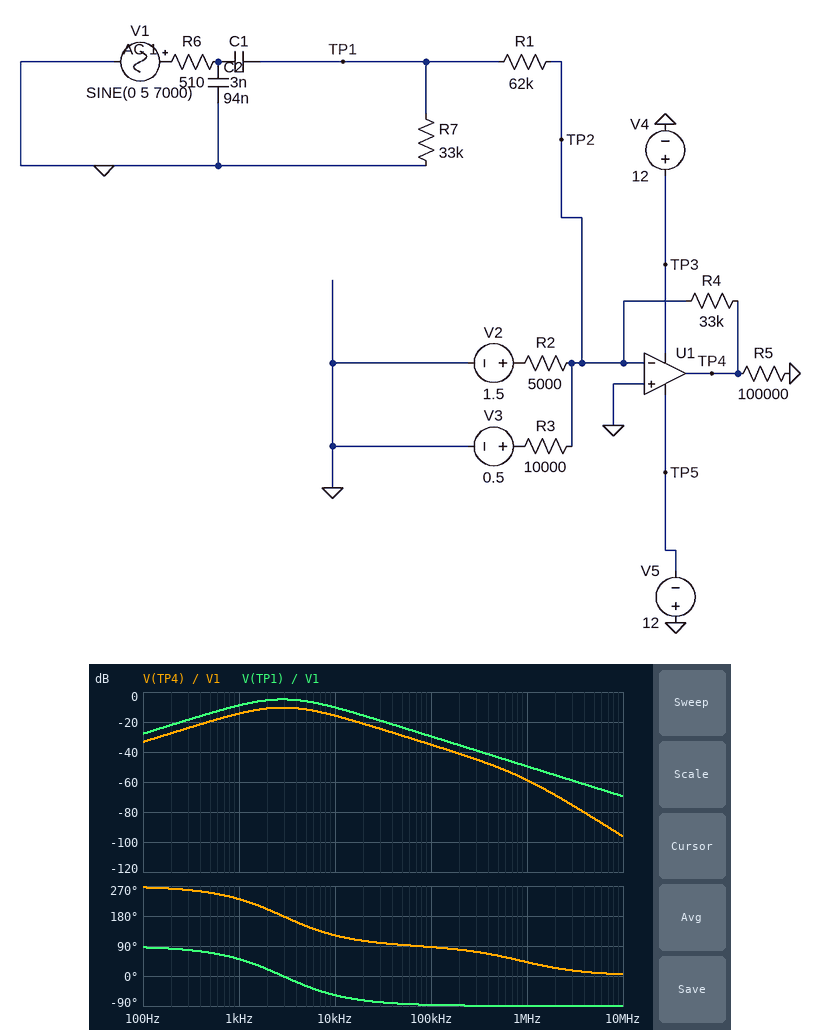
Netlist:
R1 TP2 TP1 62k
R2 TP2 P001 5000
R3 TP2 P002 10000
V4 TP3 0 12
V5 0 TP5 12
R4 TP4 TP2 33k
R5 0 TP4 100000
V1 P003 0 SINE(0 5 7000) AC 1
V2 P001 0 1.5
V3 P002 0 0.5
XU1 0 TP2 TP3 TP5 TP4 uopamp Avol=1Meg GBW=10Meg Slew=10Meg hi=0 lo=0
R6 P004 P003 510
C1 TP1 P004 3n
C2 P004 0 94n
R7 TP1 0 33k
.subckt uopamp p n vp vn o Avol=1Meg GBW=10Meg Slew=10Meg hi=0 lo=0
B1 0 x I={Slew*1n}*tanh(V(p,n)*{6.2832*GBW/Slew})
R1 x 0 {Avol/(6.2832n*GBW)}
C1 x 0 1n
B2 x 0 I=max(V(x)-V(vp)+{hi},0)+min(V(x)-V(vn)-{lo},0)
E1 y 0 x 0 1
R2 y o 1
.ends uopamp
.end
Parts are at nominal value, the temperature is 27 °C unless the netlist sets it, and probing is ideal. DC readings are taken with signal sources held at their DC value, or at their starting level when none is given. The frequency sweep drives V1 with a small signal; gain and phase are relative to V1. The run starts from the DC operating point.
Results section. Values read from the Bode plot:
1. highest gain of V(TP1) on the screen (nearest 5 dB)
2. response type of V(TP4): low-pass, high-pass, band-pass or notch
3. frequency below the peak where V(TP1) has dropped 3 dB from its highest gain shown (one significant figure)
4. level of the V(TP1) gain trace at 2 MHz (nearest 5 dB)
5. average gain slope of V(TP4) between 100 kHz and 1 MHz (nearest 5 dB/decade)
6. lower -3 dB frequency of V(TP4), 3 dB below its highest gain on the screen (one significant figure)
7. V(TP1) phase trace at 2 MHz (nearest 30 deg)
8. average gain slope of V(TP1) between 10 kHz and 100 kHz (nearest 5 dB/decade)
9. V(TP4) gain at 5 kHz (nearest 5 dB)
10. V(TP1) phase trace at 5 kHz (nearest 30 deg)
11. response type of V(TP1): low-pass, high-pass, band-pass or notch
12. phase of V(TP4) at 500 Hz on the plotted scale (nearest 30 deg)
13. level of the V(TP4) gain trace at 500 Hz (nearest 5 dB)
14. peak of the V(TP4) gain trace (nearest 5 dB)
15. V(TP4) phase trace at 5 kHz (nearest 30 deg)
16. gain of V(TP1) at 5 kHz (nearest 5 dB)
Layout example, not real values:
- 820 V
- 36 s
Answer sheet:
- -5 dB
- band-pass
- 1 kHz
- -55 dB
- -25 dB/decade
- 1 kHz
- -90 deg
- -20 dB/decade
- -10 dB
- -30 deg
- band-pass
- 240 deg
- -20 dB
- -10 dB
- 150 deg
- -5 dB
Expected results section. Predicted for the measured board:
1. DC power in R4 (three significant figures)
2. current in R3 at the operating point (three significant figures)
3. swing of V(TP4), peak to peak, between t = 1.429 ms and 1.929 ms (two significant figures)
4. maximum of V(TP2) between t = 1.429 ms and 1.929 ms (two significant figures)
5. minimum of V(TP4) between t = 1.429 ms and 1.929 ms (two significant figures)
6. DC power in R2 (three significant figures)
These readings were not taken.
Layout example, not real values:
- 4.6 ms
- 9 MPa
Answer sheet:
- 4.04 mW
- 50.0 µA
- 1.5 V
- 54 mV
- -12 V
- 450 µW
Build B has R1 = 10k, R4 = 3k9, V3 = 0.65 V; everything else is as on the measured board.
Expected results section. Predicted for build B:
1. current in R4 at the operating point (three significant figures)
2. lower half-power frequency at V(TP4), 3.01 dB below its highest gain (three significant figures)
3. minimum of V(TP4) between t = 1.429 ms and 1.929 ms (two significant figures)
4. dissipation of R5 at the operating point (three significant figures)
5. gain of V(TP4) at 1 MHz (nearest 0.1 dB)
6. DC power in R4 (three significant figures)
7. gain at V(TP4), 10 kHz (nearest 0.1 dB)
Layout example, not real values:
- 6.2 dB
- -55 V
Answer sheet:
- 365 µA
- 1.86 kHz
- -2.0 V
- 20.3 µW
- -58.0 dB
- 520 µW
- -20.0 dB
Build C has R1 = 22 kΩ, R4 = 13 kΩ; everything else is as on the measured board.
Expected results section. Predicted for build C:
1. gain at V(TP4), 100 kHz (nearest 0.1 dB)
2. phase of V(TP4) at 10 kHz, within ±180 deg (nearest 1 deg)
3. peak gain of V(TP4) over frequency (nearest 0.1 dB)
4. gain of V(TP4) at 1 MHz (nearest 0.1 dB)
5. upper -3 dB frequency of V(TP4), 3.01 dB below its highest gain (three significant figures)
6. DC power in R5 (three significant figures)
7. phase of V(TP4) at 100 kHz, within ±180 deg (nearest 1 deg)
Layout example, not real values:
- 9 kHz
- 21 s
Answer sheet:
- -34.2 dB
- 130 deg
- -11.6 dB
- -55.3 dB
- 8.96 kHz
- 207 µW
- 91 deg
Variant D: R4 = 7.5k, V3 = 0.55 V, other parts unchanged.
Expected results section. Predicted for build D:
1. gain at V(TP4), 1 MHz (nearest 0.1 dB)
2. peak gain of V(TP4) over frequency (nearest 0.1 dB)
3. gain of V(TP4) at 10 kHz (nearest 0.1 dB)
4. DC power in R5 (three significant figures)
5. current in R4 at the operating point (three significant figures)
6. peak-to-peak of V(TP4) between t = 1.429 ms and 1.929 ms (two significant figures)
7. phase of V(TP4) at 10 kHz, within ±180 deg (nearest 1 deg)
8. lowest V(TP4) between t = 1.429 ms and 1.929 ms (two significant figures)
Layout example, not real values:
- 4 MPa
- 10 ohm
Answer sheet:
- -68.4 dB
- -23.3 dB
- -28.7 dB
- 70.9 µW
- 355 µA
- 490 mV
- 122 deg
- -2.9 V
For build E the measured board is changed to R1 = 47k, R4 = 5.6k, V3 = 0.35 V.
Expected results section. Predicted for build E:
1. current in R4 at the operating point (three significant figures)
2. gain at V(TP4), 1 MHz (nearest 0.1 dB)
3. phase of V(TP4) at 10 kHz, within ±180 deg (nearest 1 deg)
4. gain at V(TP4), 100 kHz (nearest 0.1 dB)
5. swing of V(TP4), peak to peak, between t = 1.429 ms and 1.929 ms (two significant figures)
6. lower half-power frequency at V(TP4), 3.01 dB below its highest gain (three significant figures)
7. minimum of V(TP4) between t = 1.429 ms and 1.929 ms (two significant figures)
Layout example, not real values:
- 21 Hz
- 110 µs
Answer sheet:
- 335 µA
- -68.4 dB
- 124 deg
- -48.1 dB
- 470 mV
- 1.23 kHz
- -2.1 V
